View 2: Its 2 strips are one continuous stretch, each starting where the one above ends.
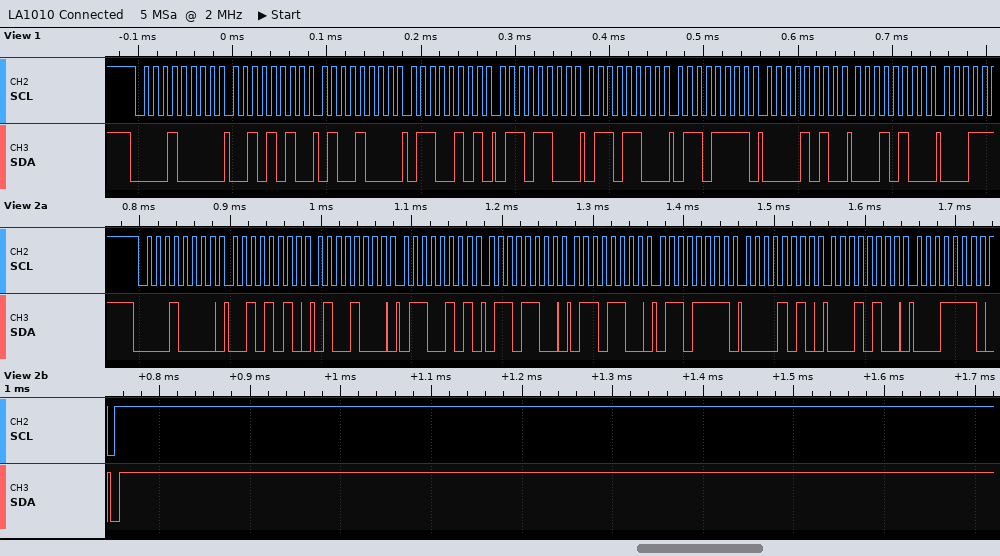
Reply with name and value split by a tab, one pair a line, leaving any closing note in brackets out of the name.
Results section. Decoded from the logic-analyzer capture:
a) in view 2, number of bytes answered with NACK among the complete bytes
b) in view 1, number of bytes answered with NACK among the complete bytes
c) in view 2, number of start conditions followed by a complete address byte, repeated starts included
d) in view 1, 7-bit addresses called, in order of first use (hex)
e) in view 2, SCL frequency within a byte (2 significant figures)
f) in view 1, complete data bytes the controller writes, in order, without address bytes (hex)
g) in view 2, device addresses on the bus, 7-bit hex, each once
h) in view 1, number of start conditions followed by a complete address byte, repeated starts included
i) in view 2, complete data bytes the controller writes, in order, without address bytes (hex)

in view 2, number of bytes answered with NACK among the complete bytes	0
in view 1, number of bytes answered with NACK among the complete bytes	0
in view 2, number of start conditions followed by a complete address byte, repeated starts included	1
in view 1, 7-bit addresses called, in order of first use	0x08
in view 2, SCL frequency within a byte	100 kHz
in view 1, complete data bytes the controller writes, in order, without address bytes	2A 48 65 6C 6C 6F 0A 14
in view 2, device addresses on the bus, 7-bit hex, each once	0x08
in view 1, number of start conditions followed by a complete address byte, repeated starts included	1
in view 2, complete data bytes the controller writes, in order, without address bytes	2A 48 65 6C 6C 6F 0A 14 1E
